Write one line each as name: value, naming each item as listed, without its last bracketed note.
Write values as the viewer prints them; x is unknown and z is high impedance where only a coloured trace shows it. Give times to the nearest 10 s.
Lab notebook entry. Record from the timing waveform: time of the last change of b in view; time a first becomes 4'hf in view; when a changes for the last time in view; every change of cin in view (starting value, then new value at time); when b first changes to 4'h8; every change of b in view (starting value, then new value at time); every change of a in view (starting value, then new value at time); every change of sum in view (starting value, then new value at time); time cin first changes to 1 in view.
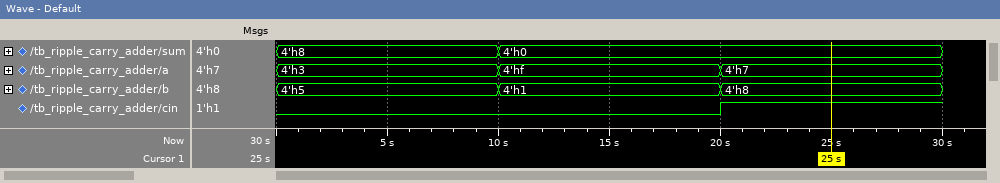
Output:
time of the last change of b in view: 20 s
time a first becomes 4'hf in view: 10 s
when a changes for the last time in view: 20 s
every change of cin in view: 0, 1 at 20 s
when b first changes to 4'h8: 20 s
every change of b in view: 4'h5, 4'h1 at 10 s, 4'h8 at 20 s
every change of a in view: 4'h3, 4'hf at 10 s, 4'h7 at 20 s
every change of sum in view: 4'h8, 4'h0 at 10 s
time cin first changes to 1 in view: 20 s
